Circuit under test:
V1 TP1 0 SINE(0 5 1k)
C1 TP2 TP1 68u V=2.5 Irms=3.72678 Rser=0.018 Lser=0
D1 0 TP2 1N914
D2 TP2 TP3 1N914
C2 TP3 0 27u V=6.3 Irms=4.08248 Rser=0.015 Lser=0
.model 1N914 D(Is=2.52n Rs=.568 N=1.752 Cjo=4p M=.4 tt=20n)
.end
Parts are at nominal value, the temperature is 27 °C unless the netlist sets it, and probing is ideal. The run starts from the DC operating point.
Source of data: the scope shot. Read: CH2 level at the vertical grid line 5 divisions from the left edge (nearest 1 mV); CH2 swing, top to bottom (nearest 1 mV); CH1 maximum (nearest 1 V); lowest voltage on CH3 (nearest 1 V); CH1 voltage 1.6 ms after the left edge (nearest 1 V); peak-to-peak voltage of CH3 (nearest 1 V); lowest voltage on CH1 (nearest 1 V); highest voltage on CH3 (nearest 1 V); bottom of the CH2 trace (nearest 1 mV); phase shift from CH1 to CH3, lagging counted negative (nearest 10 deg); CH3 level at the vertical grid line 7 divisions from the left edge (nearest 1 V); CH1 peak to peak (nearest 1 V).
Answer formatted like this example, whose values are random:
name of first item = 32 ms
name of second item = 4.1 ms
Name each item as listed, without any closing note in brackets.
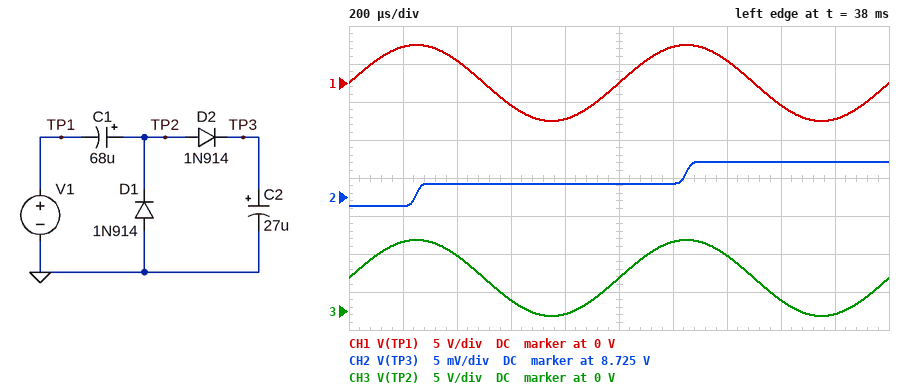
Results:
CH2 level at the vertical grid line 5 divisions from the left edge = 8.727 V
CH2 swing, top to bottom = 6 mV
CH1 maximum = 5 V
lowest voltage on CH3 = -1 V
CH1 voltage 1.6 ms after the left edge = -3 V
peak-to-peak voltage of CH3 = 10 V
lowest voltage on CH1 = -5 V
highest voltage on CH3 = 9 V
bottom of the CH2 trace = 8.724 V
phase shift from CH1 to CH3, lagging counted negative = 0 deg
CH3 level at the vertical grid line 7 divisions from the left edge = 7 V
CH1 peak to peak = 10 V
